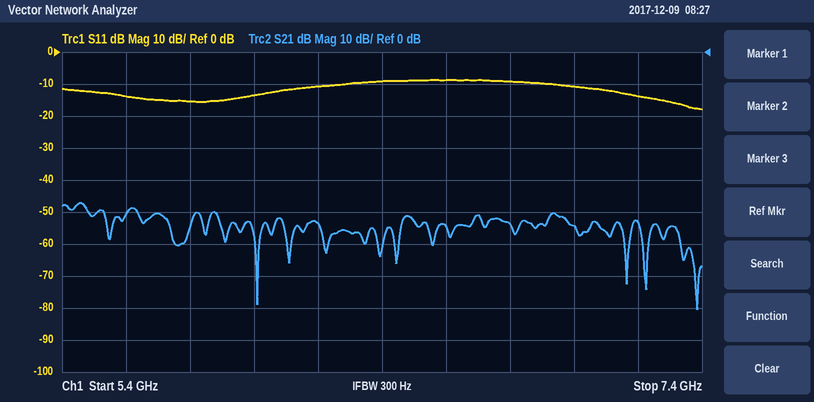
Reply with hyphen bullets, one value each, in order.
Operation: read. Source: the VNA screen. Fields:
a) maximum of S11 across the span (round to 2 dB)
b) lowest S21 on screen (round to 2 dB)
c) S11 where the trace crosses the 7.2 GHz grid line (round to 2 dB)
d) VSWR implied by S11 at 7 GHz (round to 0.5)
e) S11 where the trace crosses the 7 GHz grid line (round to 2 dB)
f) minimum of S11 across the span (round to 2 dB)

- -8 dB
- -80 dB
- -14 dB
- 2.0
- -10 dB
- -18 dB
